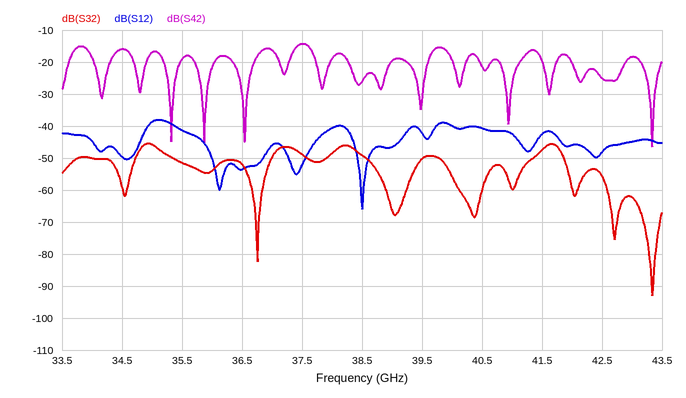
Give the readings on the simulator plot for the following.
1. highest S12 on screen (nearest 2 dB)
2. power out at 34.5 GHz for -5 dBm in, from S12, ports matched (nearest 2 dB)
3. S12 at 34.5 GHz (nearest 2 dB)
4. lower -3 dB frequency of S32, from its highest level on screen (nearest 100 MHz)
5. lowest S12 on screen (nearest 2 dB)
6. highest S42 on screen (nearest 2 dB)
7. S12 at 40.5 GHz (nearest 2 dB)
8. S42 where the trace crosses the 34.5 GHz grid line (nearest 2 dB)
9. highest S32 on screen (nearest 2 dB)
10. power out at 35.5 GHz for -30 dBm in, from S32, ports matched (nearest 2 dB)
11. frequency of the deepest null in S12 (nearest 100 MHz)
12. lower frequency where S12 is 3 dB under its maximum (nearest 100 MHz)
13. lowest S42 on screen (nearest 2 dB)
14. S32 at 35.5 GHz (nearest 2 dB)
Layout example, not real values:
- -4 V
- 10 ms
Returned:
- -38 dB
- -54 dBm
- -50 dB
- 34.8 GHz
- -66 dB
- -14 dB
- -40 dB
- -16 dB
- -46 dB
- -82 dBm
- 38.5 GHz
- 34.9 GHz
- -46 dB
- -52 dB
